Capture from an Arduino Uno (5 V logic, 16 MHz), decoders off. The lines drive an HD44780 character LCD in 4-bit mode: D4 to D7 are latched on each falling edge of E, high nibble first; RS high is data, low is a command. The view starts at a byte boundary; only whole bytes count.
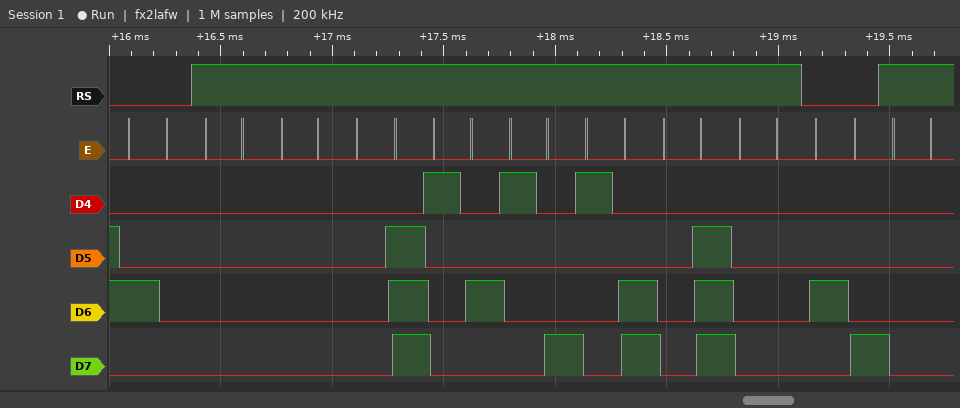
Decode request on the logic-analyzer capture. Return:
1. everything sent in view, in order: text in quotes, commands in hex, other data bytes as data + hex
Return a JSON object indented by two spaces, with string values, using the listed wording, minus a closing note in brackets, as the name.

{
  "everything sent in view, in order: text in quotes, commands in hex, other data bytes as data + hex": "0x40 data 00 00 0E 14 18 1C 0E 00 0x48 data 00"
}
